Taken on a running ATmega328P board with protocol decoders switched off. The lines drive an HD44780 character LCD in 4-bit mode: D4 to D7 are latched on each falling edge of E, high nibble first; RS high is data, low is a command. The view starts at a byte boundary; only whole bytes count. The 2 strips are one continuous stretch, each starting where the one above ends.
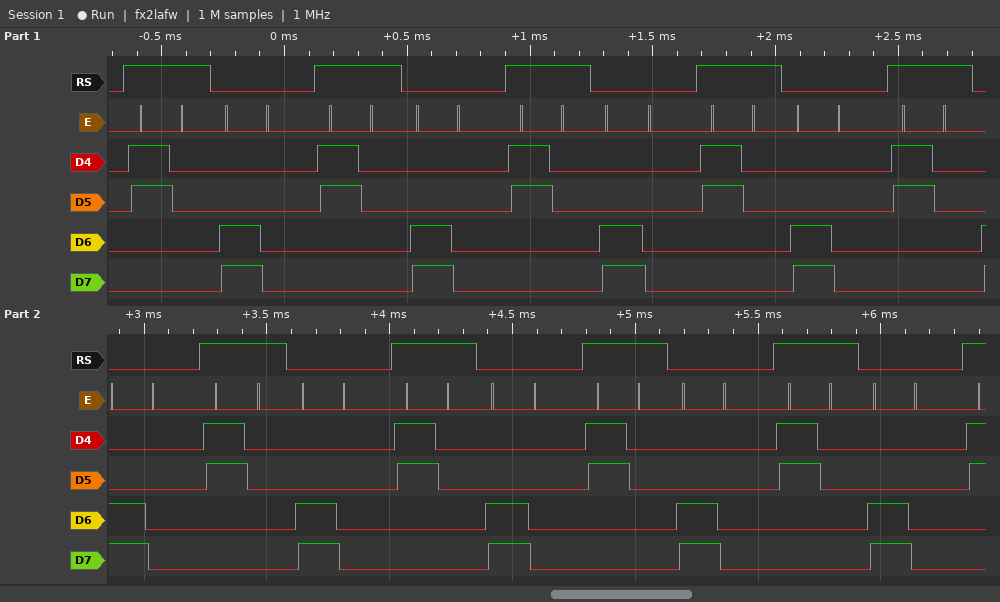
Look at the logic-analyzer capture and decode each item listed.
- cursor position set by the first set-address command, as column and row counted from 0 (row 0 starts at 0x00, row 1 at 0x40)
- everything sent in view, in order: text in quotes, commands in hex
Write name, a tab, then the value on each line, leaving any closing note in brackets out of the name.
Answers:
cursor position set by the first set-address command, as column and row counted from 0	column 0, row 1
everything sent in view, in order: text in quotes, commands in hex	"0" 0xC0 "0" 0xC0 "0" 0xC0 "0" 0xC0 "0" 0xC0 "0" 0xC0 "0" 0xC0 "0" 0xC0 "0" 0xC0
